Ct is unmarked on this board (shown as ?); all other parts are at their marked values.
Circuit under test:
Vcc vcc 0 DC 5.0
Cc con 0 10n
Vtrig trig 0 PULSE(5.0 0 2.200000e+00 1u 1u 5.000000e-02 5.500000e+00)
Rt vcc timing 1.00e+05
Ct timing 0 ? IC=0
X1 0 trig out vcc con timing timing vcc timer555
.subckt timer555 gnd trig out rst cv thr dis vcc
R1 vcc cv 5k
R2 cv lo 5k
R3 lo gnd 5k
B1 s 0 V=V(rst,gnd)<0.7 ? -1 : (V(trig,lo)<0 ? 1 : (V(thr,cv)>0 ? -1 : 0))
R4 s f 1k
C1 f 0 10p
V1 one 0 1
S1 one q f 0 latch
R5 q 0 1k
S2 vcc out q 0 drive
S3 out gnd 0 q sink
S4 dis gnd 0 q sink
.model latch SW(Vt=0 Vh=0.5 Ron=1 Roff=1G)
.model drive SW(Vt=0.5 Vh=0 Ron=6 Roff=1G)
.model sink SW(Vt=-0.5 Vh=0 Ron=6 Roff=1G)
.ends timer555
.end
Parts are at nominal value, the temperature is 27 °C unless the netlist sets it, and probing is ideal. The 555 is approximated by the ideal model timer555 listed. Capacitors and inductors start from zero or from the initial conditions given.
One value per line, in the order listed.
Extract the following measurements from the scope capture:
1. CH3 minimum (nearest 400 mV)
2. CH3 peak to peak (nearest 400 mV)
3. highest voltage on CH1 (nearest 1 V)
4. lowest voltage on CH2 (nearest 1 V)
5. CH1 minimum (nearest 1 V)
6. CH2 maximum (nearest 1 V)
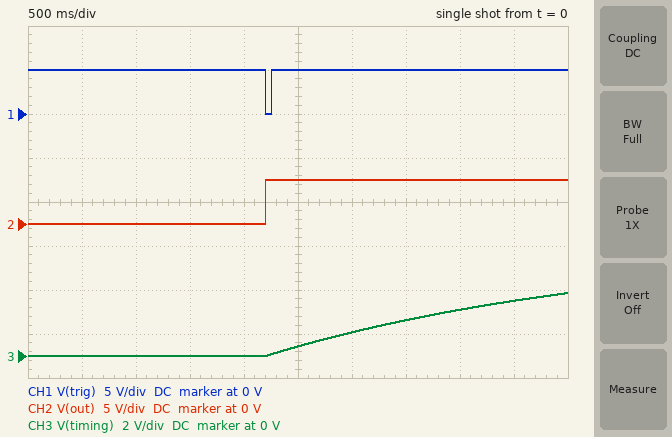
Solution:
0 V
2.8 V
5 V
0 V
0 V
5 V
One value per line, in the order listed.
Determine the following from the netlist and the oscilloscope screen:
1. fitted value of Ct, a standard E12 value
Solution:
33 µF
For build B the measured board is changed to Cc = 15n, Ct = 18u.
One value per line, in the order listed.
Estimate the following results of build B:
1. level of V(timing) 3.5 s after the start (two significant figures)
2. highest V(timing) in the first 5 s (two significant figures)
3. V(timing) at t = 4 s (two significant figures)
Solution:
2.6 V
3.3 V
3.2 V
